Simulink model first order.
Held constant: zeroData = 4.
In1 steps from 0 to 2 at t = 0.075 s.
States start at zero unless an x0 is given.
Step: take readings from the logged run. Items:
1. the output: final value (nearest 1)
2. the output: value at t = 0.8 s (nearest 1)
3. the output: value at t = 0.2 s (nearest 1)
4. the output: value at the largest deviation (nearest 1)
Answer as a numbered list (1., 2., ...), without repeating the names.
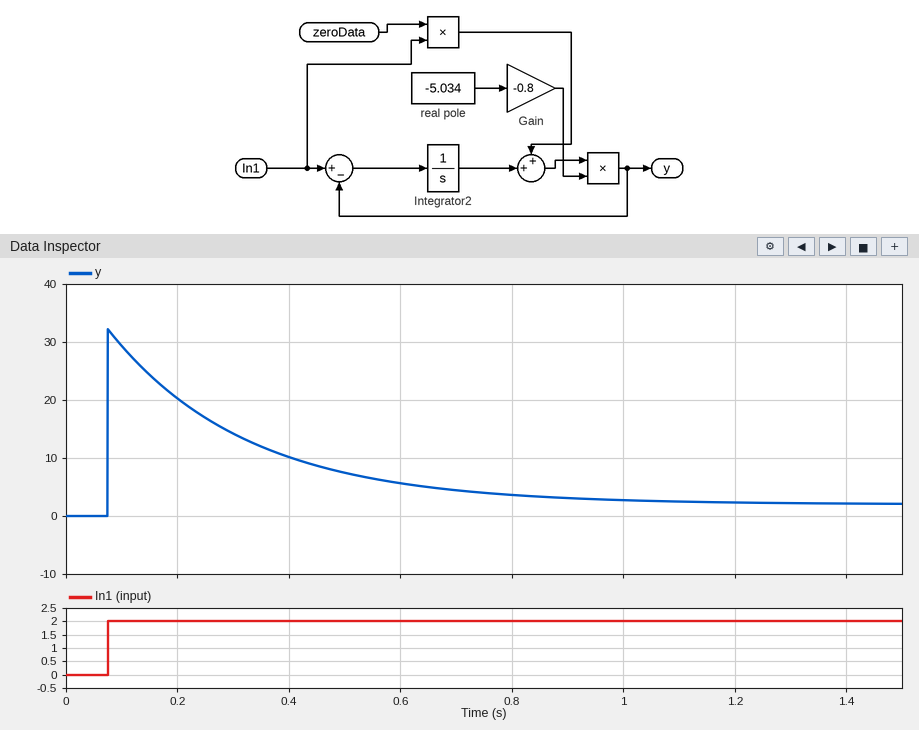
1. 2
2. 4
3. 20
4. 32
